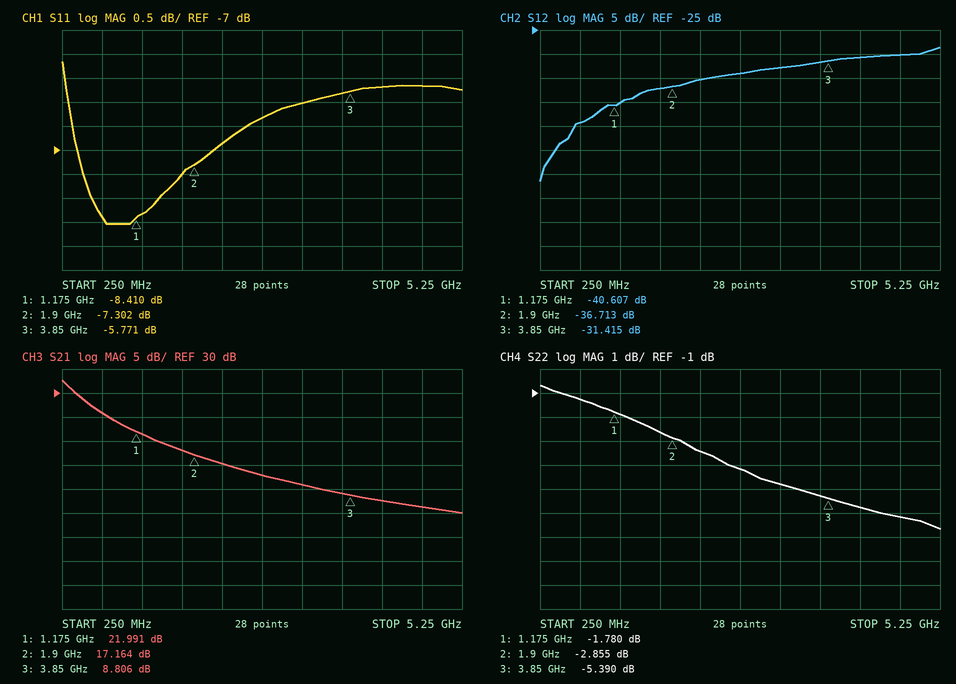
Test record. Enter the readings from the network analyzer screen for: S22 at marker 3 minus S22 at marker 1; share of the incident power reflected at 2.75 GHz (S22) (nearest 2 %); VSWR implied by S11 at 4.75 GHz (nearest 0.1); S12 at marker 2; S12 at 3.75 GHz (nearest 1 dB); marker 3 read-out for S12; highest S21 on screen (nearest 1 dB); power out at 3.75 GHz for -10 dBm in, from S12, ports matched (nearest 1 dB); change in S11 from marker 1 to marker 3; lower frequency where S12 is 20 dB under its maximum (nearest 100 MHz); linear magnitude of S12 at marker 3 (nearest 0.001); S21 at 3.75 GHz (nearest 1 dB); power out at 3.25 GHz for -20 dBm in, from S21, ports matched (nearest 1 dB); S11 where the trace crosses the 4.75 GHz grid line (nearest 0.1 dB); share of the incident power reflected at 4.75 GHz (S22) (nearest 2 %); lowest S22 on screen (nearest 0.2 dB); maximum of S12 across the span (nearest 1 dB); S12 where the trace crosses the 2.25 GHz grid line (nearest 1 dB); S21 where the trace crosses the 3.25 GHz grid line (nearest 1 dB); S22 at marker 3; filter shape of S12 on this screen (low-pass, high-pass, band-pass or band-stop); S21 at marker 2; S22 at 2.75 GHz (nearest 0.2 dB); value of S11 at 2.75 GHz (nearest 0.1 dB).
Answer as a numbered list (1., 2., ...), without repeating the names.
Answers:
1. -3.610 dB
2. 38 %
3. 3.2
4. -36.713 dB
5. -32 dB
6. -31.415 dB
7. 33 dB
8. -42 dBm
9. 2.639 dB
10. 500 MHz
11. 0.027
12. 9 dB
13. -9 dBm
14. -5.7 dB
15. 24 %
16. -6.6 dB
17. -29 dB
18. -35 dB
19. 11 dB
20. -5.390 dB
21. high-pass
22. 17.164 dB
23. -4.2 dB
24. -6.3 dB
